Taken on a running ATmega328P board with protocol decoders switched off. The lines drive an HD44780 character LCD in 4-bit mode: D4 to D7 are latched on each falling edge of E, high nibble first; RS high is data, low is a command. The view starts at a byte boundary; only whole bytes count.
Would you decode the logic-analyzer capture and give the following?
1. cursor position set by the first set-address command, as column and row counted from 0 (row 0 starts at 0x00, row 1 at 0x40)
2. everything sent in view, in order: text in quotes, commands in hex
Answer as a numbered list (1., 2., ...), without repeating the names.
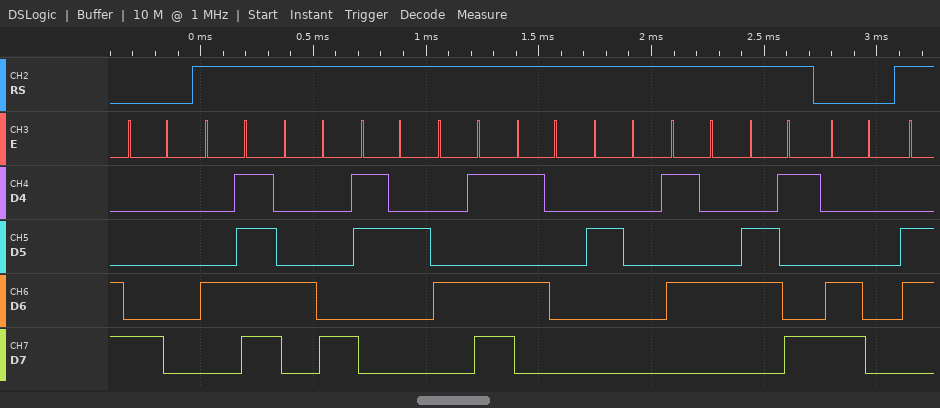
1. column 0, row 0
2. 0x80 "OH2MP Ti" 0xC0
